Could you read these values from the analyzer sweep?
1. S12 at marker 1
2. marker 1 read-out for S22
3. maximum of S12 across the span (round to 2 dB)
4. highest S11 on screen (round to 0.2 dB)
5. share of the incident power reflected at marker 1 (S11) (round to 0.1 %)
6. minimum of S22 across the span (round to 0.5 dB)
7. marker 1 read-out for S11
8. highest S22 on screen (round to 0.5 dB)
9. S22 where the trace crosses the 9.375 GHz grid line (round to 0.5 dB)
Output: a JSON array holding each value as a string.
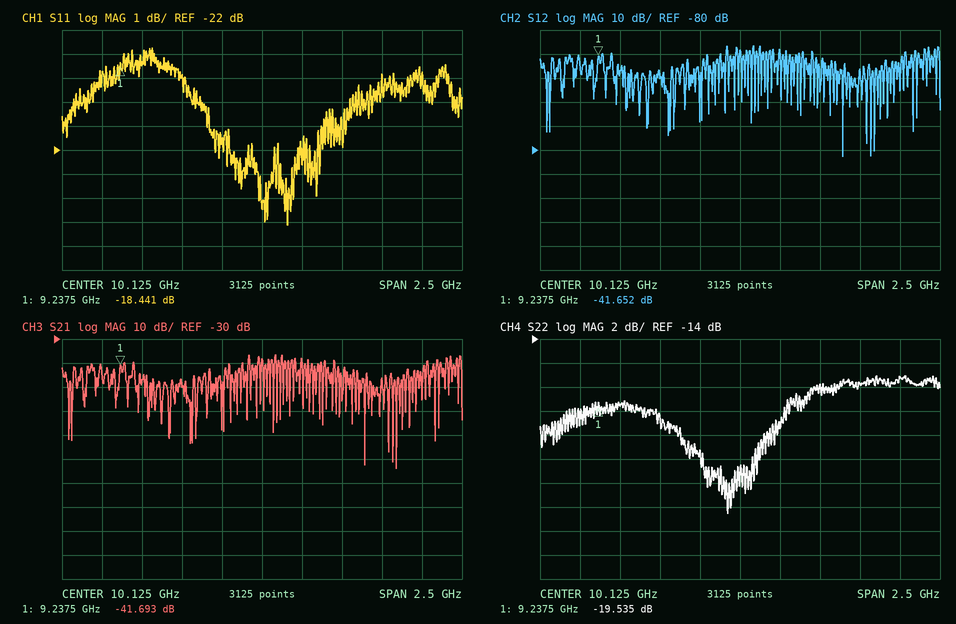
["-41.652 dB", "-19.535 dB", "-36 dB", "-17.8 dB", "1.4 %", "-28.5 dB", "-18.441 dB", "-17.0 dB", "-19.5 dB"]
